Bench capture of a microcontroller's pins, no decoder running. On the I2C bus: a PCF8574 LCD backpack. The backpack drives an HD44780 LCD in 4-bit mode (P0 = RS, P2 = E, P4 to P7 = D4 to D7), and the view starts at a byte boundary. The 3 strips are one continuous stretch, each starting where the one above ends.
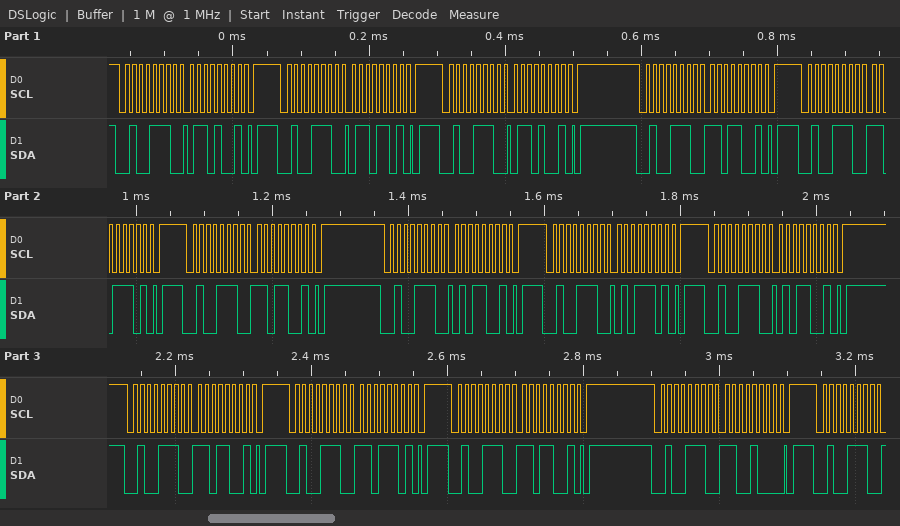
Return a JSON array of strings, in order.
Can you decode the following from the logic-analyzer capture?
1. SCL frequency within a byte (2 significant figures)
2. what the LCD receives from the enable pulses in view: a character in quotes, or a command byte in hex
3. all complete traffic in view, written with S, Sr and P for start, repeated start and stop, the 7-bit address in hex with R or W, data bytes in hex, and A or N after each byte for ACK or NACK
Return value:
["100 kHz", "'m' ']'", "S 27W A 69 A P S 27W A 6D A P S 27W A 69 A P S 27W A D9 A P S 27W A DD A P S 27W A D9 A P S 27W A 59 A P S 27W A 5D A P S 27W A 59 A P S 27W A D9 A P S 27W A DD A P S 27W A D9 A P S 27W A C8 A P S 27W A"]
